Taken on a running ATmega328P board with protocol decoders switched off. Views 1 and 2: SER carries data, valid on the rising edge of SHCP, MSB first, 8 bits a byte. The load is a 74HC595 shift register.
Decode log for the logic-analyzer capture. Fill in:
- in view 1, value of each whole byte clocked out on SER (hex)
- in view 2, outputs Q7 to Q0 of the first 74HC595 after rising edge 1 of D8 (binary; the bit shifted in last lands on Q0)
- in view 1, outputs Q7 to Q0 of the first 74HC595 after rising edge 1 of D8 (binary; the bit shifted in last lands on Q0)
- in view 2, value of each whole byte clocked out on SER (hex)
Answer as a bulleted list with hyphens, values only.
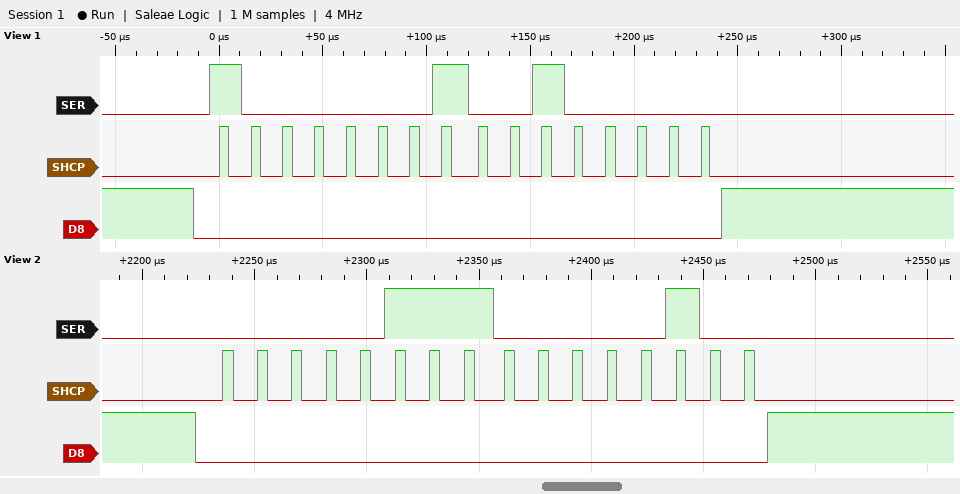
- 81 20
- 00000100
- 00100000
- 07 04
